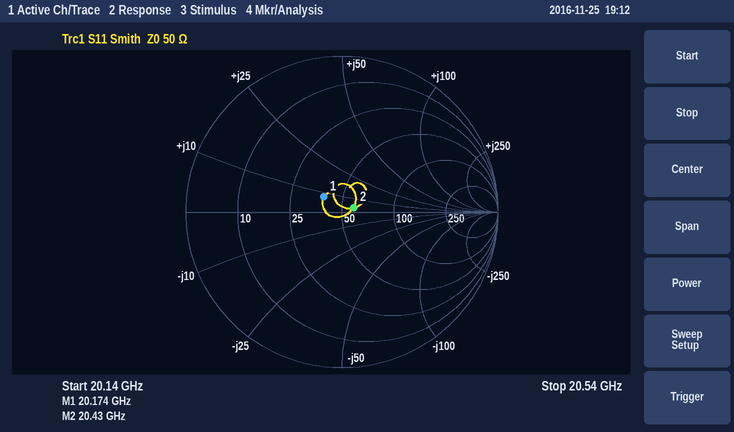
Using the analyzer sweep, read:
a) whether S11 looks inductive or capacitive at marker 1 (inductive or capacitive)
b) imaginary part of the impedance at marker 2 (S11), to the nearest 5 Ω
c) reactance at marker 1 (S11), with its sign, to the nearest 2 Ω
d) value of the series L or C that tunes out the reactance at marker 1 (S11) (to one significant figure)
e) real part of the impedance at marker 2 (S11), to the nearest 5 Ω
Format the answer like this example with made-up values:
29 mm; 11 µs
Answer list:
inductive; +5 Ω; +8 Ω; 1 pF; 60 Ω
